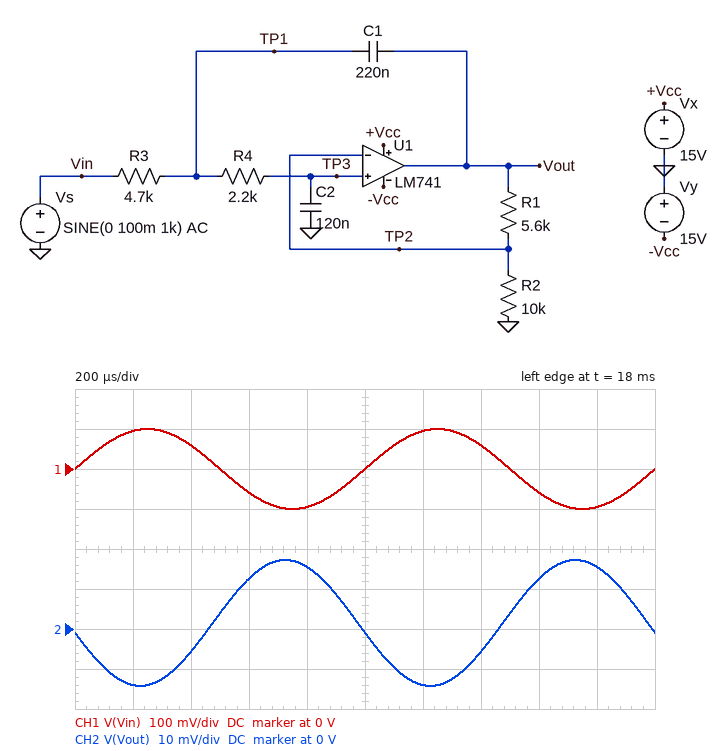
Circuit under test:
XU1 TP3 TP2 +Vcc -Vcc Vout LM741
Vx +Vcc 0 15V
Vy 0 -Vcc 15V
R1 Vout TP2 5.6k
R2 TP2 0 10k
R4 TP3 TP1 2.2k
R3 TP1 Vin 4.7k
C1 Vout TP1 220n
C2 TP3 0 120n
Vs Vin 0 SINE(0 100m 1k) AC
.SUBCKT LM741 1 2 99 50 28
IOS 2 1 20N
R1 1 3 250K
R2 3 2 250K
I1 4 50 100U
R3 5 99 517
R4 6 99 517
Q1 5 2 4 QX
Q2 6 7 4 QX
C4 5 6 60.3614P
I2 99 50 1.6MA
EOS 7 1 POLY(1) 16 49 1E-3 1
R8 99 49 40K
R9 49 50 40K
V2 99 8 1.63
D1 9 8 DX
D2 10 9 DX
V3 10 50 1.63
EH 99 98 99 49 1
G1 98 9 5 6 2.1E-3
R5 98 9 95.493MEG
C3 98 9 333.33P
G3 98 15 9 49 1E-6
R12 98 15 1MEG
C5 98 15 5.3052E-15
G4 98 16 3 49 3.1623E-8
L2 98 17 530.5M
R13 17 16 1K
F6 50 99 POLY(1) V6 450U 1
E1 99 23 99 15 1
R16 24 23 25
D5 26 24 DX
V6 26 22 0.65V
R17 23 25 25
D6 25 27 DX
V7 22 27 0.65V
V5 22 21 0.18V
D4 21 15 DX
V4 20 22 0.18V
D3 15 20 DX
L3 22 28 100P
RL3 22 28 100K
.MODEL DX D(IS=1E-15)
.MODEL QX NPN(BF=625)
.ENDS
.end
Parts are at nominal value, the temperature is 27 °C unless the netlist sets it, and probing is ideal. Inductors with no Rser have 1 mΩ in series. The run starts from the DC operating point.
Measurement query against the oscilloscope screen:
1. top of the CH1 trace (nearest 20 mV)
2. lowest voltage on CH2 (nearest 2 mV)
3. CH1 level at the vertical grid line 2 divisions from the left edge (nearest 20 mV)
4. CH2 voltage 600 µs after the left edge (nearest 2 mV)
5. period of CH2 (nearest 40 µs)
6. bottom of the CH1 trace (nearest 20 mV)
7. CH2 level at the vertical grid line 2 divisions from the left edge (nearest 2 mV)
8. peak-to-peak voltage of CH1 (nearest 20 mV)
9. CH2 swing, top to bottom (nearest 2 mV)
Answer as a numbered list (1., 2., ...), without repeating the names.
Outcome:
1. 100 mV
2. -14 mV
3. 60 mV
4. 12 mV
5. 1.00 ms
6. -100 mV
7. -6 mV
8. 200 mV
9. 32 mV
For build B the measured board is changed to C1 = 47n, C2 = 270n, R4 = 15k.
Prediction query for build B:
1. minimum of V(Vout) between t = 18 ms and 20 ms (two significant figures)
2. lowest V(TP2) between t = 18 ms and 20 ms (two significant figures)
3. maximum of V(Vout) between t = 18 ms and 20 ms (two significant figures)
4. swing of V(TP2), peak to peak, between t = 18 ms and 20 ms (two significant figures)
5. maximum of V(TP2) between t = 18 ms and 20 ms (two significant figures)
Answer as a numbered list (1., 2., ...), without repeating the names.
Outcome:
1. -2.8 mV
2. -2.2 mV
3. 3.8 mV
4. 4.2 mV
5. 2.1 mV
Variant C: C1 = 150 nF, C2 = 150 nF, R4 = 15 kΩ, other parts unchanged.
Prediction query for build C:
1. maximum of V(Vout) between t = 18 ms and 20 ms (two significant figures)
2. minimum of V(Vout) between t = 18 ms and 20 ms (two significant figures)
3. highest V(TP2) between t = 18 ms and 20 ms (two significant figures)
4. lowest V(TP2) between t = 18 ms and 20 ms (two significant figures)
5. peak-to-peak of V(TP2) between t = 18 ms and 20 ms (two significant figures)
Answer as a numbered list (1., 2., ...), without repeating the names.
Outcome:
1. 2.8 mV
2. -2.1 mV
3. 1.4 mV
4. -1.7 mV
5. 3.1 mV
